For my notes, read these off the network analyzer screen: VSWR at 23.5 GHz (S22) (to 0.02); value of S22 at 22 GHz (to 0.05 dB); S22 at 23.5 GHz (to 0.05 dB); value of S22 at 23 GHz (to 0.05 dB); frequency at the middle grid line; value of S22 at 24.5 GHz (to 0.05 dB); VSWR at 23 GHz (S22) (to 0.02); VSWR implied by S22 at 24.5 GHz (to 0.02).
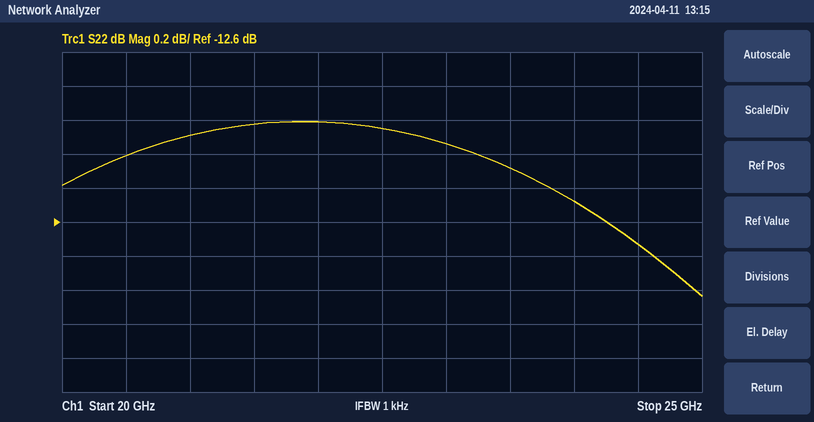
1.64
-12.00 dB
-12.30 dB
-12.15 dB
22.5 GHz
-12.75 dB
1.66
1.60
